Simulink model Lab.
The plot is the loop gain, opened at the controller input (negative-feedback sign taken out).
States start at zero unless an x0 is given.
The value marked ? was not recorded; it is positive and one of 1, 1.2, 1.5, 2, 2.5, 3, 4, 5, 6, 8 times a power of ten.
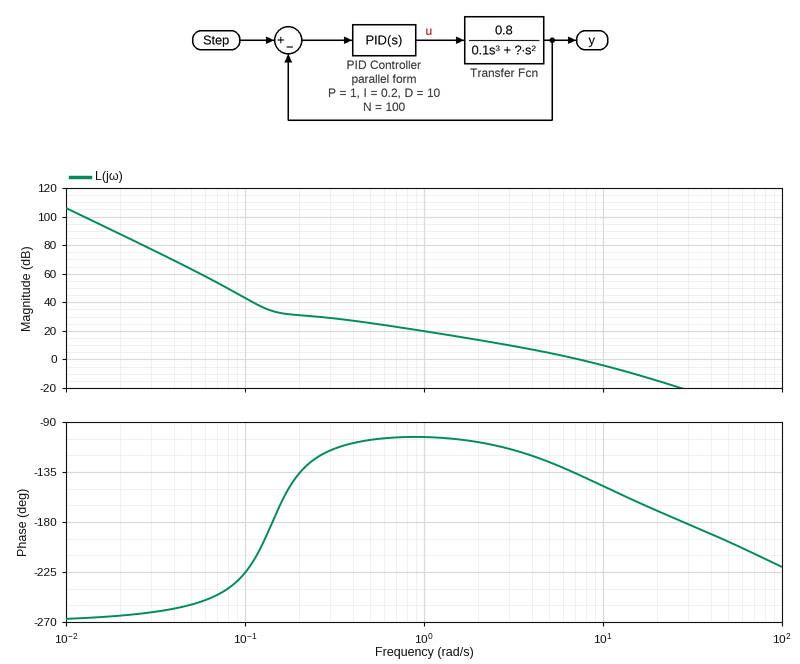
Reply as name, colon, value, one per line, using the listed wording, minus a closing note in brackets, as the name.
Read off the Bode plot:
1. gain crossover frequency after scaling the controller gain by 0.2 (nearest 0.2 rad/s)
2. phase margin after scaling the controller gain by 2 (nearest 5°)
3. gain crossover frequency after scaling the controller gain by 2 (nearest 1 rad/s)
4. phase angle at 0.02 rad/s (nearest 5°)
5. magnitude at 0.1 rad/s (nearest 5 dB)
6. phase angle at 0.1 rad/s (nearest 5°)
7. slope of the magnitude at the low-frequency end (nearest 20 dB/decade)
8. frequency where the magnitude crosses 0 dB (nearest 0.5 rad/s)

gain crossover frequency after scaling the controller gain by 0.2: 2.0 rad/s
phase margin after scaling the controller gain by 2: 30°
gain crossover frequency after scaling the controller gain by 2: 11 rad/s
phase angle at 0.02 rad/s: -265°
magnitude at 0.1 rad/s: 45 dB
phase angle at 0.1 rad/s: -225°
slope of the magnitude at the low-frequency end: -60 dB/decade
frequency where the magnitude crosses 0 dB: 7.5 rad/s
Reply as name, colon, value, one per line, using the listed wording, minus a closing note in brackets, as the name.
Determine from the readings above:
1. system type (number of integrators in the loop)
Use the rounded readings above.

system type: 3
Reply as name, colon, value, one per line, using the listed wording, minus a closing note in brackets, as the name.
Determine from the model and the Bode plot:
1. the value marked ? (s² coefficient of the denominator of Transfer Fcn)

the value marked ?: 0.8
